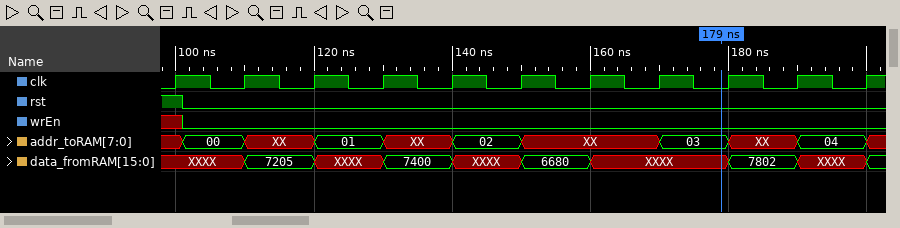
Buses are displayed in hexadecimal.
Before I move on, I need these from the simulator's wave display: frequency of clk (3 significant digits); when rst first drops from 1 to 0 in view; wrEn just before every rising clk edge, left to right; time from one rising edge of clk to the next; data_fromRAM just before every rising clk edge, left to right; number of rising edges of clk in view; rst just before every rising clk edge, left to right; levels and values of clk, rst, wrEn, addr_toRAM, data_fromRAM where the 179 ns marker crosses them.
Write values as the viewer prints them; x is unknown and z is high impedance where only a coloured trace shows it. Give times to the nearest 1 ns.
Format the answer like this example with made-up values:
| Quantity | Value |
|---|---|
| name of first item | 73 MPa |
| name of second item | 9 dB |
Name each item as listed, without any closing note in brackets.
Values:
| Quantity | Value |
|---|---|
| frequency of clk | 100 MHz |
| when rst first drops from 1 to 0 in view | 101 ns |
| wrEn just before every rising clk edge, left to right | x 0 0 0 0 0 0 0 0 0 0 |
| time from one rising edge of clk to the next | 10 ns |
| data_fromRAM just before every rising clk edge, left to right | XXXX, XXXX, 7205, XXXX, 7400, XXXX, 6680, XXXX, XXXX, 7802, XXXX |
| number of rising edges of clk in view | 11 |
| rst just before every rising clk edge, left to right | 1 0 0 0 0 0 0 0 0 0 0 |
| levels and values of clk, rst, wrEn, addr_toRAM, data_fromRAM where the 179 ns marker crosses them | clk=0, rst=0, wrEn=0, addr_toRAM=03, data_fromRAM=XXXX |
